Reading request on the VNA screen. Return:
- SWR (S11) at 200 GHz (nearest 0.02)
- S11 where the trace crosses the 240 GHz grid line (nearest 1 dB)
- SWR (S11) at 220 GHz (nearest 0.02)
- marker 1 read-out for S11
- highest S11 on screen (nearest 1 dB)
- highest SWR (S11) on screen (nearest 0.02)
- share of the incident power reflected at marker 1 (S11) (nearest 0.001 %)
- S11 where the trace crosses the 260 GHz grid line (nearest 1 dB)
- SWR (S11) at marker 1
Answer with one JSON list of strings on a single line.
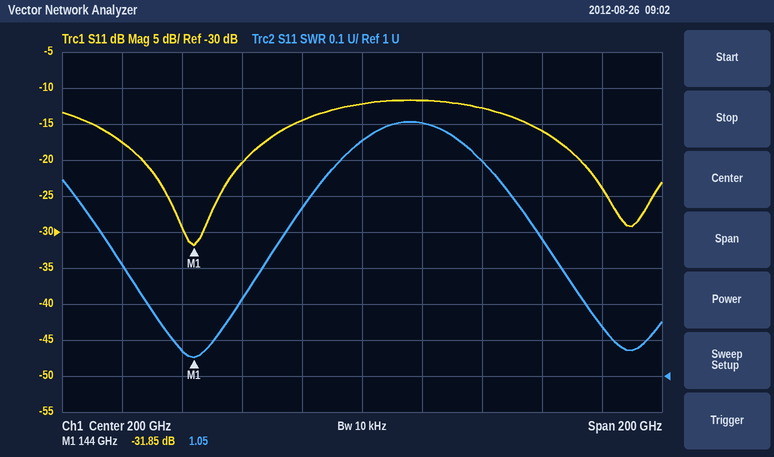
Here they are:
["1.66", "-13 dB", "1.70", "-31.85 dB", "-12 dB", "1.70", "0.065 %", "-16 dB", "1.05"]
